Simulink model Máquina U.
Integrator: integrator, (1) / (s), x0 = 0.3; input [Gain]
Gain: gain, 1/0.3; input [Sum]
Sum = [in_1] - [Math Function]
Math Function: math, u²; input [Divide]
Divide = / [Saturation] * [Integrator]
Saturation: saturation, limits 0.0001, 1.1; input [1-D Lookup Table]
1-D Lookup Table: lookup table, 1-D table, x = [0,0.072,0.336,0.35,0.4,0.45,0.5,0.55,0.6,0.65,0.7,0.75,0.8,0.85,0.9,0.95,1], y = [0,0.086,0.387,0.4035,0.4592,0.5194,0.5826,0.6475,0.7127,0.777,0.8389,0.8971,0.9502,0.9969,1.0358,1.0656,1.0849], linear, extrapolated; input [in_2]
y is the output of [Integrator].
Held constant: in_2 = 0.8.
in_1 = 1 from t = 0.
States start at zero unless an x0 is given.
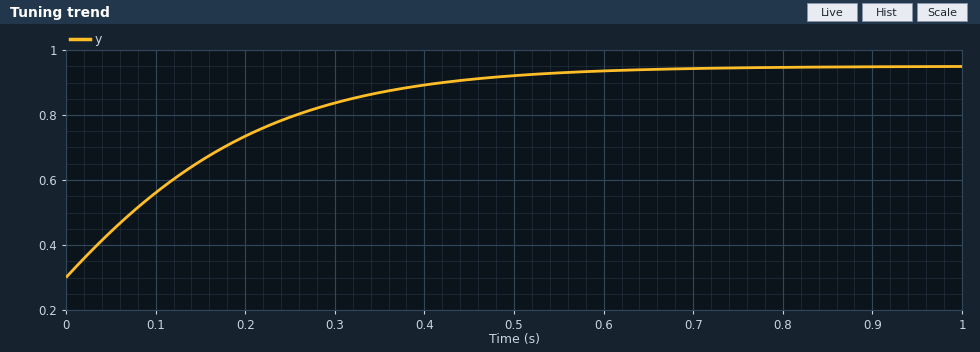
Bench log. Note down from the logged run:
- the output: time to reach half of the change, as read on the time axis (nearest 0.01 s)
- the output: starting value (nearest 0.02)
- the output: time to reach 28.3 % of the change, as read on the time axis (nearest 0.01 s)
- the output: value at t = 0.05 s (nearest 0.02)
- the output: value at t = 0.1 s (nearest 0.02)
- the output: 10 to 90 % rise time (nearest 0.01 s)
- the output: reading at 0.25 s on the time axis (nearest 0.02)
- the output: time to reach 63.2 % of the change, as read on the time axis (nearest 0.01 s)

0.13 s
0.30
0.07 s
0.44
0.56
0.36 s
0.80
0.18 s
